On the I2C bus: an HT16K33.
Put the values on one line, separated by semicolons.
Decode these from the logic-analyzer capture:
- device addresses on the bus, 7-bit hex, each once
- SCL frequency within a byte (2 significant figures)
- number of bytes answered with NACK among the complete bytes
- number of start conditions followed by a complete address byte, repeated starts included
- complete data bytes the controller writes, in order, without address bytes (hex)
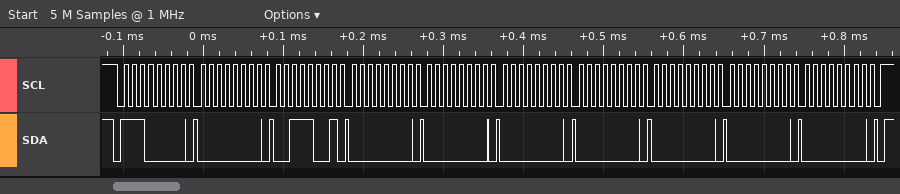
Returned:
0x70; 100 kHz; 0; 1; 00 39 00 00 00 00 00 00 00
